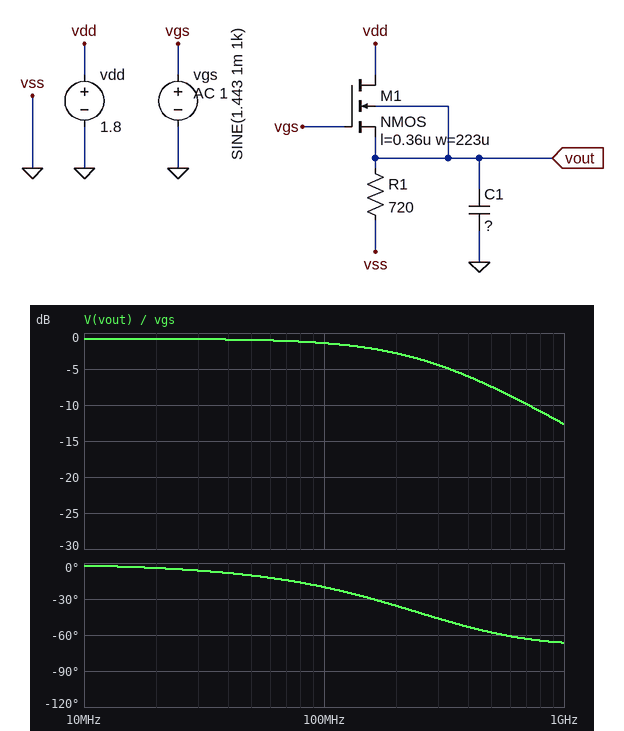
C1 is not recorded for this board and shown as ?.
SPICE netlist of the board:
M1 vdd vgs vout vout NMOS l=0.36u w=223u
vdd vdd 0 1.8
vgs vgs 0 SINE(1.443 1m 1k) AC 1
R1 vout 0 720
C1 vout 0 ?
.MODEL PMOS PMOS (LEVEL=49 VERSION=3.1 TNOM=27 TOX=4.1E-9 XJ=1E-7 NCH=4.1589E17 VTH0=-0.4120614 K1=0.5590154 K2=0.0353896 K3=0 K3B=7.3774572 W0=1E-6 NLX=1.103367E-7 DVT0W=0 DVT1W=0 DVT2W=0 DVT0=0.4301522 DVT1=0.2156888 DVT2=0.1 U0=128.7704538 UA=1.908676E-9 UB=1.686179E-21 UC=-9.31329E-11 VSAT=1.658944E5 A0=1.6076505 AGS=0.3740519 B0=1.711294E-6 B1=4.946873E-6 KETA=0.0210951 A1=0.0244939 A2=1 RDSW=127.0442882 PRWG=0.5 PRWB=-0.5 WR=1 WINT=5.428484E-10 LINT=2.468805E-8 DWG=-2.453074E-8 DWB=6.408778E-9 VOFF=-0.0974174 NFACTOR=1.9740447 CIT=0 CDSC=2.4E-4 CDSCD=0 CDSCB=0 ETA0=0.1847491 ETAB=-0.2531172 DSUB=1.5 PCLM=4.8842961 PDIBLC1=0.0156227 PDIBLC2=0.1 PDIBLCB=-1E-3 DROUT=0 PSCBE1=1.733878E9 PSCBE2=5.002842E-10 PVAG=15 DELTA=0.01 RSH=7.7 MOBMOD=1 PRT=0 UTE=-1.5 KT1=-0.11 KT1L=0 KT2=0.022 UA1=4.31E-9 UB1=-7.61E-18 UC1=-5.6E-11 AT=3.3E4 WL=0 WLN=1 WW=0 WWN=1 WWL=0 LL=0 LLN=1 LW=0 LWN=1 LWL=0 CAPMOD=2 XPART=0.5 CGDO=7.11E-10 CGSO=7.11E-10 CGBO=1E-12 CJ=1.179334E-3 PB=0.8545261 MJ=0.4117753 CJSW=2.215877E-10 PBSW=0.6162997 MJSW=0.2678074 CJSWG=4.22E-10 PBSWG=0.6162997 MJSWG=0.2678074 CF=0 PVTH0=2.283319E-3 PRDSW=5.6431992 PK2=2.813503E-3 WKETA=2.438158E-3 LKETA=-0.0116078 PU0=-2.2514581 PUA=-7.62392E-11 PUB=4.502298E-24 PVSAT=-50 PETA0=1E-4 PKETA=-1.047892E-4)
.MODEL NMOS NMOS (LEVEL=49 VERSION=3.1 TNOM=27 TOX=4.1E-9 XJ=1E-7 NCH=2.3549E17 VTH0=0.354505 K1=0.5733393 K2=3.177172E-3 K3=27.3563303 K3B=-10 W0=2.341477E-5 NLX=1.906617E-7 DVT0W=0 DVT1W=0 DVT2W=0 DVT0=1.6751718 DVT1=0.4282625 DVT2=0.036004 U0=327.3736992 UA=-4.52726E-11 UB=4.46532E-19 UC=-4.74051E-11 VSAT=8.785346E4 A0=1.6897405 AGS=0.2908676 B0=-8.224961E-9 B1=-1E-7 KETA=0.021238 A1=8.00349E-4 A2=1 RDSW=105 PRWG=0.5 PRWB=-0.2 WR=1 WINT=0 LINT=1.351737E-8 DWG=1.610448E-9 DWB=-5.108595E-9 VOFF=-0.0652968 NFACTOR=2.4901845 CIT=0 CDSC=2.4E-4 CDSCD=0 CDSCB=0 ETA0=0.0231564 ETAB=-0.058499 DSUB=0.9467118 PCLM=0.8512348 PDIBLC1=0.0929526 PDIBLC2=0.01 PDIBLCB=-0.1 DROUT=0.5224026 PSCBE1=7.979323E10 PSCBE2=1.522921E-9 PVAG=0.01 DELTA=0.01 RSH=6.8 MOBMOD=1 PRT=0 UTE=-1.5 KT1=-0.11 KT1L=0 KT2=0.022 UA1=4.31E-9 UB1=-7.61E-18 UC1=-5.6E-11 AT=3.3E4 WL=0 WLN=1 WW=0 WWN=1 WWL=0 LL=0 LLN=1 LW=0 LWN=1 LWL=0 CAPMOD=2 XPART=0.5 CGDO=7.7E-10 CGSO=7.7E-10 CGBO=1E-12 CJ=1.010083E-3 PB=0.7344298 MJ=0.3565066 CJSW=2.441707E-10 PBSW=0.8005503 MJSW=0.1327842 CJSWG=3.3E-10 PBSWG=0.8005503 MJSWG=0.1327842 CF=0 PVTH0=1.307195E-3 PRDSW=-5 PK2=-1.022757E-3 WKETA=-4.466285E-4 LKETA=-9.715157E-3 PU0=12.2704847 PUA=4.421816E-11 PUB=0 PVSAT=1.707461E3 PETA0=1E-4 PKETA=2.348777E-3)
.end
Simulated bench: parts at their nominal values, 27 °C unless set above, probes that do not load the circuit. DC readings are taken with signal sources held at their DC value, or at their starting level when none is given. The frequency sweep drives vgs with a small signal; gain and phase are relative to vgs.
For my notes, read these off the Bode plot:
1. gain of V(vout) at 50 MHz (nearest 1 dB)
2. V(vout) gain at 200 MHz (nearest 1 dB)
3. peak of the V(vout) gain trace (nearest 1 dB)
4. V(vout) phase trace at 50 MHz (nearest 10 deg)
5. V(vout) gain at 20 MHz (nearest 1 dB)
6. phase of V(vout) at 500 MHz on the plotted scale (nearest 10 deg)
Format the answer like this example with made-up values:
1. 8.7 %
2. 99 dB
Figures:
1. -1 dB
2. -3 dB
3. -1 dB
4. -10 deg
5. -1 dB
6. -60 deg
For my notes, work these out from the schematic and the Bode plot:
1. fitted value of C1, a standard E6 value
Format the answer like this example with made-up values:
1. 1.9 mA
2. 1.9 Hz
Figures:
1. 10 pF
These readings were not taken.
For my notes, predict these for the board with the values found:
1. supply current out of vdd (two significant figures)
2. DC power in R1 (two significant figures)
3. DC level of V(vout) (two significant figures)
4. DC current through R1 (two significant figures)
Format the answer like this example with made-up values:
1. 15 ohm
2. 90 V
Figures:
1. 1.2 mA
2. 960 µW
3. 830 mV
4. 1.2 mA
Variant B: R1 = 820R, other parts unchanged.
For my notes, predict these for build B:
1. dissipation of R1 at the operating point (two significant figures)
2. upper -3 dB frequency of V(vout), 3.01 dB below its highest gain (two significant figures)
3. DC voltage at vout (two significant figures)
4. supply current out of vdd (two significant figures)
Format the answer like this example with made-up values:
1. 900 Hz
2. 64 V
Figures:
1. 860 µW
2. 240 MHz
3. 840 mV
4. 1.0 mA
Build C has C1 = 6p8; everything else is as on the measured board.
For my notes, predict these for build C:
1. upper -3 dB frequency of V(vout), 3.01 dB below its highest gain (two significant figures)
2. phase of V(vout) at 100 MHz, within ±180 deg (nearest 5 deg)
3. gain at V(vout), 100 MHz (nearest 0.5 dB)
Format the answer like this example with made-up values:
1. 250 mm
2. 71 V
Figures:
1. 380 MHz
2. -15 deg
3. -1.0 dB
